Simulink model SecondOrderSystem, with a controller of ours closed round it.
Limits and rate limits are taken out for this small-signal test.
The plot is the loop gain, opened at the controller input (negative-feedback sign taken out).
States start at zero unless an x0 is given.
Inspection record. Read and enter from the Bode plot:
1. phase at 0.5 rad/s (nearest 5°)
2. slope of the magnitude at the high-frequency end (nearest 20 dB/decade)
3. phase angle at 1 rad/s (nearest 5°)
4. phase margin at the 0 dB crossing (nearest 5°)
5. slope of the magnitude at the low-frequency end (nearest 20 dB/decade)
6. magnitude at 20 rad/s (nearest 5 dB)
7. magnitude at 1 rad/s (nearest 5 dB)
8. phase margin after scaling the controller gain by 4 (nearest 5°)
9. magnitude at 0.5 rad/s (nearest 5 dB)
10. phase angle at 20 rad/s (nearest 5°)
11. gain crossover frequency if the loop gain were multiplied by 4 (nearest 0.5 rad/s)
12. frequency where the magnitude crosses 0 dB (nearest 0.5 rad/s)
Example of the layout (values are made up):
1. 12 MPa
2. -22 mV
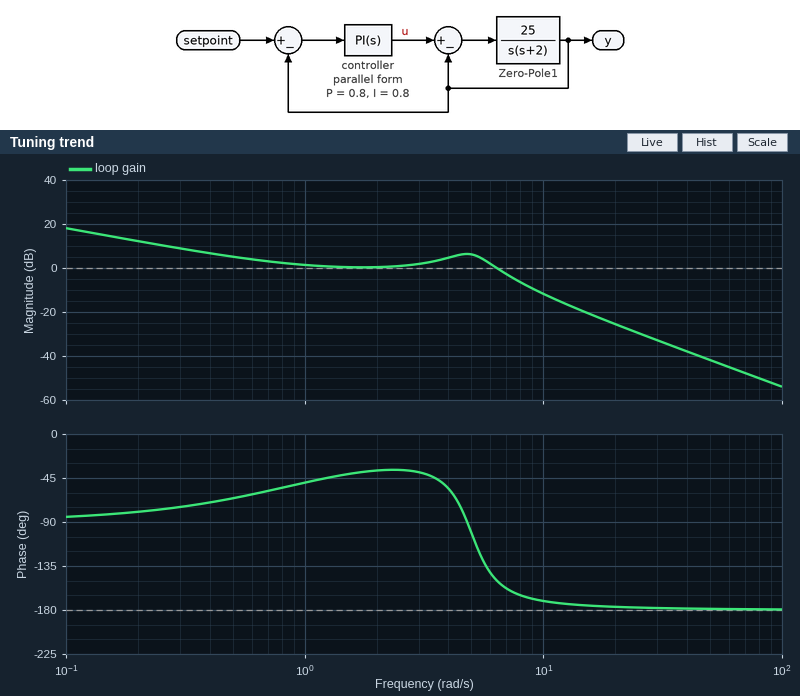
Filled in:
1. -65°
2. -40 dB/decade
3. -50°
4. 30°
5. -20 dB/decade
6. -25 dB
7. 0 dB
8. 10°
9. 5 dB
10. -175°
11. 10.0 rad/s
12. 6.5 rad/s
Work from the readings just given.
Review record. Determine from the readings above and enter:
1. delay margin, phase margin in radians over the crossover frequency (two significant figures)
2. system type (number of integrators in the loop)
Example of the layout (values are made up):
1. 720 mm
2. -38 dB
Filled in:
1. 0.081 s
2. 1
